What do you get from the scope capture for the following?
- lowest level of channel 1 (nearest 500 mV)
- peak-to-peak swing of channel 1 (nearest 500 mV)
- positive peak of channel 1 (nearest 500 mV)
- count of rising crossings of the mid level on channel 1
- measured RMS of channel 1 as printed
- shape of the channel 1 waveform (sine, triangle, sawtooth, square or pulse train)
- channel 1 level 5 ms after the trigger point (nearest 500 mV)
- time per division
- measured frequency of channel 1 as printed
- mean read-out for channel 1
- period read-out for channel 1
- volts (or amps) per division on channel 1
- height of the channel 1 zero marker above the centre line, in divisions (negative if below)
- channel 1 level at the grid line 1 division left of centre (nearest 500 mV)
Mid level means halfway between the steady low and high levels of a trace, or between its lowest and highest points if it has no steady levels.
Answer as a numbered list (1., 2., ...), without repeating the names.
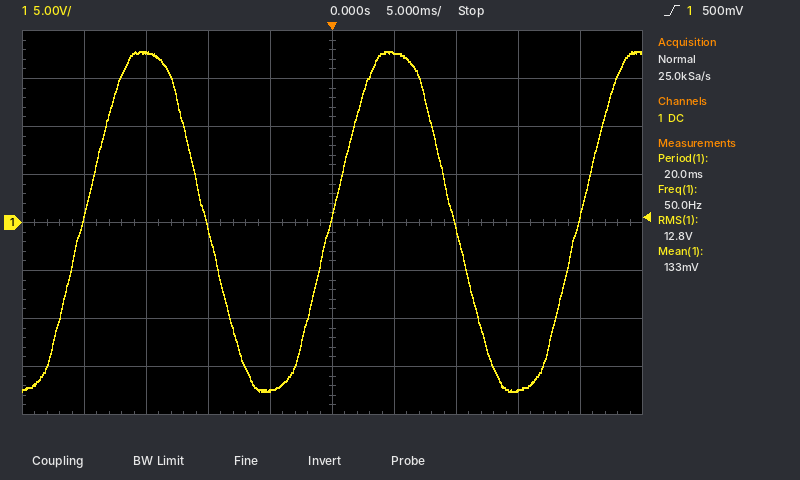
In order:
1. -17.5 V
2. 35.5 V
3. 18.0 V
4. 3
5. 12.8 V
6. sine
7. 17.5 V
8. 5 ms
9. 50.0 Hz
10. 133 mV
11. 20.0 ms
12. 5 V
13. 0.0 div
14. -17.5 V
